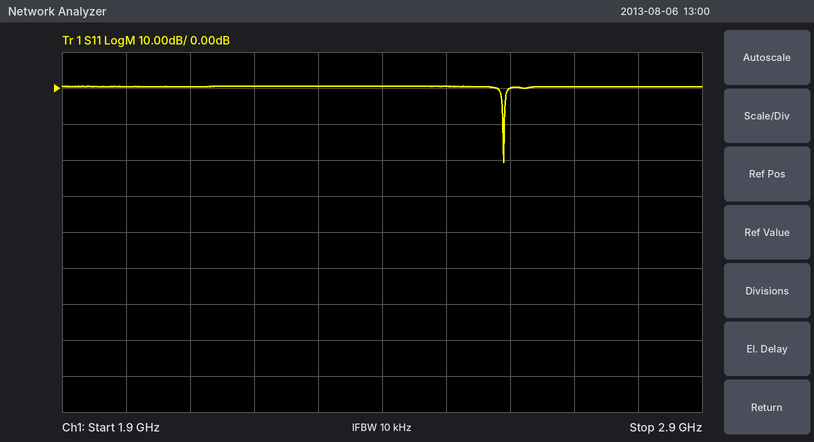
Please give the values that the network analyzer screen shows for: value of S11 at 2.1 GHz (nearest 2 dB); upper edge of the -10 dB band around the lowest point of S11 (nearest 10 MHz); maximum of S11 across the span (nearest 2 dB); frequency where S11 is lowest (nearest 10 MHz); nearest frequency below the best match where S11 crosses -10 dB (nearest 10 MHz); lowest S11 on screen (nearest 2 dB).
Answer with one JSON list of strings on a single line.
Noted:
["0 dB", "2.59 GHz", "0 dB", "2.59 GHz", "2.59 GHz", "-20 dB"]
